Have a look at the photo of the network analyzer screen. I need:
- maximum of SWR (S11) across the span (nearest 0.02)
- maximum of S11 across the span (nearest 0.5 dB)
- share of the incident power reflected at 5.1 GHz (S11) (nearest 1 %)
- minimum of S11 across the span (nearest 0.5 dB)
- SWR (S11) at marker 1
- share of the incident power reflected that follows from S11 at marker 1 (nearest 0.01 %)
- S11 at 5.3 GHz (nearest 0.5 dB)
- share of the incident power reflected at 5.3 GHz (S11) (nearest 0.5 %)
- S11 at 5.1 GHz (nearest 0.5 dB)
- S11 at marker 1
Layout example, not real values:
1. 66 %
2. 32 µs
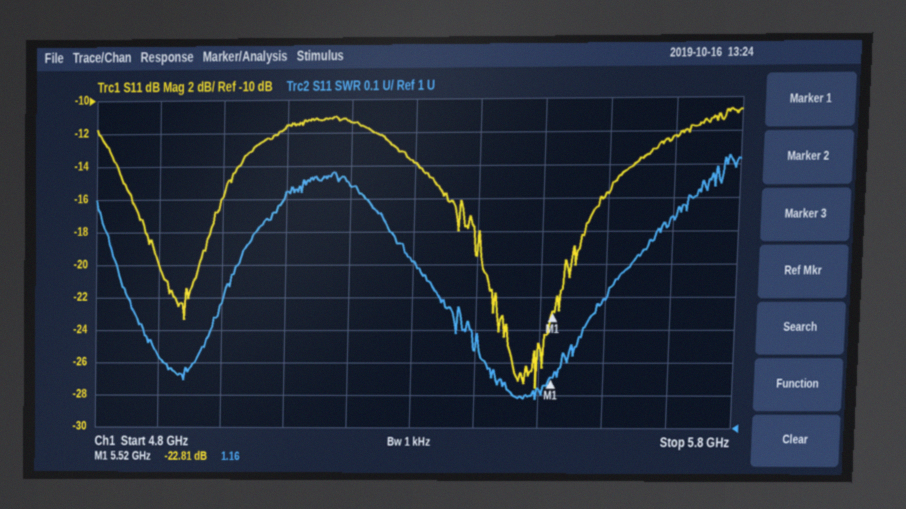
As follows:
1. 1.82
2. -10.5 dB
3. 7 %
4. -27.5 dB
5. 1.16
6. 0.52 %
7. -14.0 dB
8. 4.0 %
9. -11.5 dB
10. -22.81 dB
